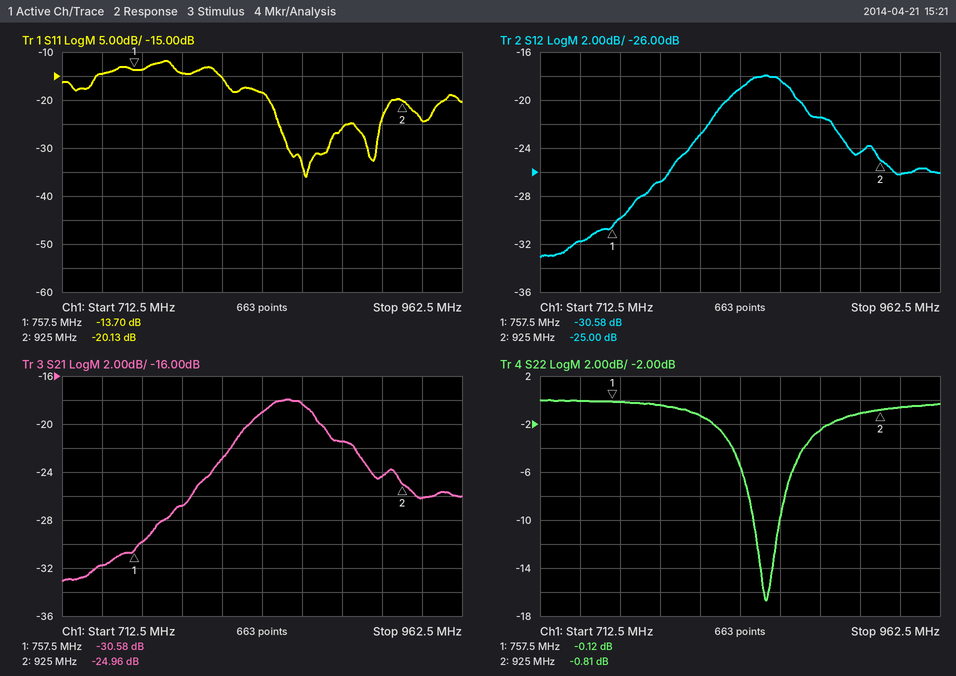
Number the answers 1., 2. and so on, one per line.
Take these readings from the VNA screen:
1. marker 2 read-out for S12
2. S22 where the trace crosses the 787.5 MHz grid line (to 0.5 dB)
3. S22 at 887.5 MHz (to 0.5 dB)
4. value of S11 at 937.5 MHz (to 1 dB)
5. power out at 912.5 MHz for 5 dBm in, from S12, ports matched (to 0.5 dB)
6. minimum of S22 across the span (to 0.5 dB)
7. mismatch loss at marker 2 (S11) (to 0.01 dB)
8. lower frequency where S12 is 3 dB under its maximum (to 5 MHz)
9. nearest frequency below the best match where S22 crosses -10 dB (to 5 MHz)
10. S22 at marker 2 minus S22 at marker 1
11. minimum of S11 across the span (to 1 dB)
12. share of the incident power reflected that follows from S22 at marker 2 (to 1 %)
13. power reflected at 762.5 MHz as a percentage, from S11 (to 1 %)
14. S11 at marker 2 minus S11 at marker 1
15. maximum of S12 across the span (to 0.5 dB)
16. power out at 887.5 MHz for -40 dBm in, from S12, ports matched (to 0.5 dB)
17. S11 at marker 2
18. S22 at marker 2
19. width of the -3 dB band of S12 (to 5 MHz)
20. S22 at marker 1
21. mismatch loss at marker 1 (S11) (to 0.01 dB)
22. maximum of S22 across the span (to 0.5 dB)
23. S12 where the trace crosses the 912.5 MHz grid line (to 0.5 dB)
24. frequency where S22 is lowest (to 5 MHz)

1. -25.00 dB
2. -0.5 dB
3. -2.5 dB
4. -24 dB
5. -19.5 dBm
6. -16.5 dB
7. 0.04 dB
8. 825 MHz
9. 845 MHz
10. -0.69 dB
11. -36 dB
12. 83 %
13. 4 %
14. -6.43 dB
15. -18.0 dB
16. -61.5 dBm
17. -20.13 dB
18. -0.81 dB
19. 55 MHz
20. -0.12 dB
21. 0.19 dB
22. 0.0 dB
23. -24.5 dB
24. 855 MHz
